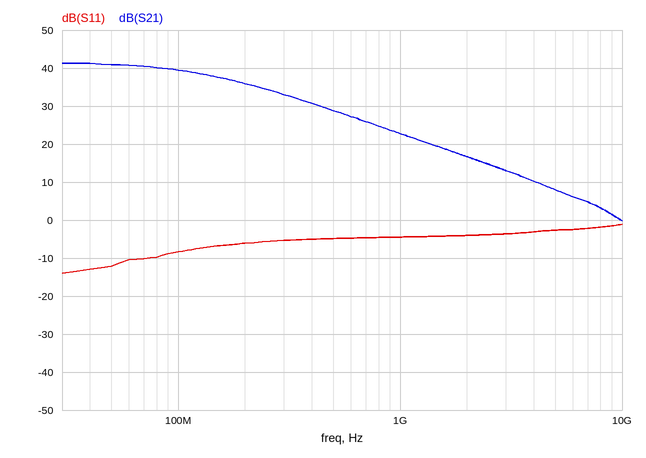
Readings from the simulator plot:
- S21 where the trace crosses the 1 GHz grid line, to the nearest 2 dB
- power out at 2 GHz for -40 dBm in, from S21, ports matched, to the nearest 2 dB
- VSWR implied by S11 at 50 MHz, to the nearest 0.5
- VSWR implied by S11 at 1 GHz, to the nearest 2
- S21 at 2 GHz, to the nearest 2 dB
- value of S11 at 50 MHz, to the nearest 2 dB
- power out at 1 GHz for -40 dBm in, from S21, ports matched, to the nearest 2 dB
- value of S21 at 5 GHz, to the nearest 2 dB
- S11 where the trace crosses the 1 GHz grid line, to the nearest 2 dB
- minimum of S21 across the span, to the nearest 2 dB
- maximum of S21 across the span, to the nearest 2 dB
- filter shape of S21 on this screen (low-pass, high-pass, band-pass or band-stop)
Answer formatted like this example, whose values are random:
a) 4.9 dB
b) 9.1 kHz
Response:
a) 22 dB
b) -24 dBm
c) 1.5
d) 4
e) 16 dB
f) -12 dB
g) -18 dBm
h) 8 dB
i) -4 dB
j) 0 dB
k) 42 dB
l) low-pass
